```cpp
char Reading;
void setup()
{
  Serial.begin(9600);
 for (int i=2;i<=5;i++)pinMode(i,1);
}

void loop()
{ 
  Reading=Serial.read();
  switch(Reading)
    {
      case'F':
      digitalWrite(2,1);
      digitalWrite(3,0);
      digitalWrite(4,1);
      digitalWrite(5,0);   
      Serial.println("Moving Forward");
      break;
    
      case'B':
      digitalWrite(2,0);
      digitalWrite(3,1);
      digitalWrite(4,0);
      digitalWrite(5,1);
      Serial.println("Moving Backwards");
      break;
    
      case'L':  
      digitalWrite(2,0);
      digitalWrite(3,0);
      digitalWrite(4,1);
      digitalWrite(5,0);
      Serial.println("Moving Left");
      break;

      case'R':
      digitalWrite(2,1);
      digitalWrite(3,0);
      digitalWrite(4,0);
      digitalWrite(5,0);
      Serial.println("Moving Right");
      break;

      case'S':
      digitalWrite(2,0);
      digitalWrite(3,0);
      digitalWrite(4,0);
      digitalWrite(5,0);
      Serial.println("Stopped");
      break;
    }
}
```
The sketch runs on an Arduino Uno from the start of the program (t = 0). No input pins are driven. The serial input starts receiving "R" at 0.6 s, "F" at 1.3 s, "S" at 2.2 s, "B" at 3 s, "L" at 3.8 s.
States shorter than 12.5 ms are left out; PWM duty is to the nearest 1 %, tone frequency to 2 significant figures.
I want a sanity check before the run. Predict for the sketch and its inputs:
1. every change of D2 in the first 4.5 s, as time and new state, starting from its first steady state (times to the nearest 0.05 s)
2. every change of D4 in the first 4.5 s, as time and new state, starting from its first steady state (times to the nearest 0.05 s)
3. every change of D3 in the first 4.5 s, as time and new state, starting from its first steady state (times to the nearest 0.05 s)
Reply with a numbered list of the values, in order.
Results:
1. 0 s low; 0.6 s high; 2.2 s low
2. 0 s low; 1.3 s high; 2.2 s low; 3.8 s high
3. 0 s low; 3 s high; 3.8 s low
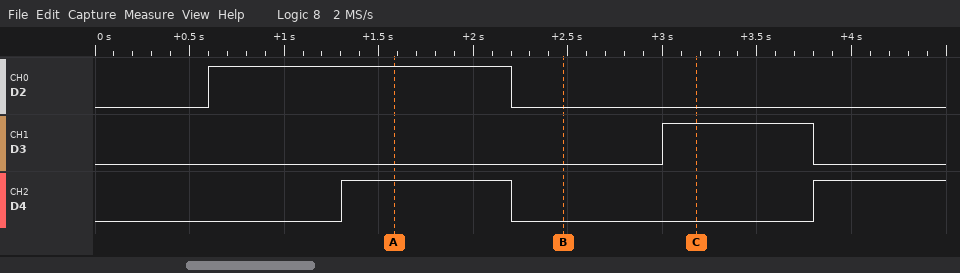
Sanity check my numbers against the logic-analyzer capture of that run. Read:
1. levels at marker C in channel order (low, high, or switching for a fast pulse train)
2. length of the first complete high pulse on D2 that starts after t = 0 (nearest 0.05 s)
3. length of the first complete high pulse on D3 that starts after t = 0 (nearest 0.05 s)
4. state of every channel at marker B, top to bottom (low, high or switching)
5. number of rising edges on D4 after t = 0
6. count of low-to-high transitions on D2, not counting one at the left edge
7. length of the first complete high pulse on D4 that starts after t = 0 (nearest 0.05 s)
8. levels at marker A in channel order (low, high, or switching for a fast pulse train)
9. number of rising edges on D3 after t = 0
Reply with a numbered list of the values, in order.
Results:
1. D2 low, D3 high, D4 low
2. 1.60 s
3. 0.80 s
4. D2 low, D3 low, D4 low
5. 2
6. 1
7. 0.90 s
8. D2 high, D3 low, D4 high
9. 1
